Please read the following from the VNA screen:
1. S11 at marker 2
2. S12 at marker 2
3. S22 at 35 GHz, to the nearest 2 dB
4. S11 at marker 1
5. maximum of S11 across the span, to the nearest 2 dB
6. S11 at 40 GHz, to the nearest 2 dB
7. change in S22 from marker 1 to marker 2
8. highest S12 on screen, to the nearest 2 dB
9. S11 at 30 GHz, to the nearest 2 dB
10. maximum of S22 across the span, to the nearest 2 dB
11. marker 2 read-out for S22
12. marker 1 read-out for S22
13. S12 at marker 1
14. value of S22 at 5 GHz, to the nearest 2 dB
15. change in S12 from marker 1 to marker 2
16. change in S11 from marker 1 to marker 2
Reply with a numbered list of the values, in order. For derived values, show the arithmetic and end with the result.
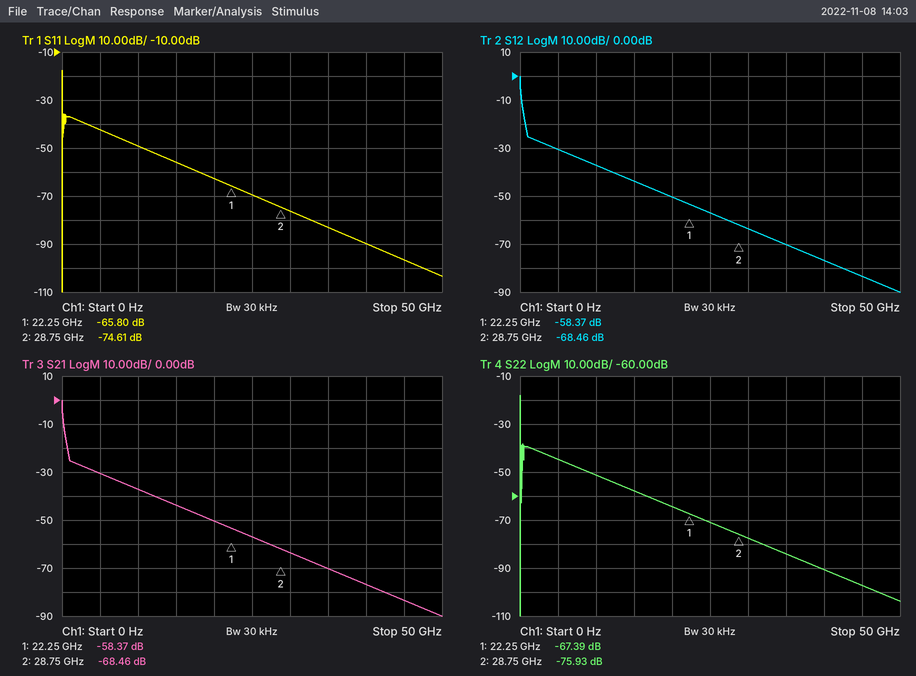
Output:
1. -74.61 dB
2. -68.46 dB
3. -84 dB
4. -65.80 dB
5. -18 dB
6. -90 dB
7. -75.93 − (-67.39) = -8.54 dB
8. 0 dB
9. -76 dB
10. -18 dB
11. -75.93 dB
12. -67.39 dB
13. -58.37 dB
14. -44 dB
15. -68.46 − (-58.37) = -10.09 dB
16. -74.61 − (-65.8) = -8.81 dB
